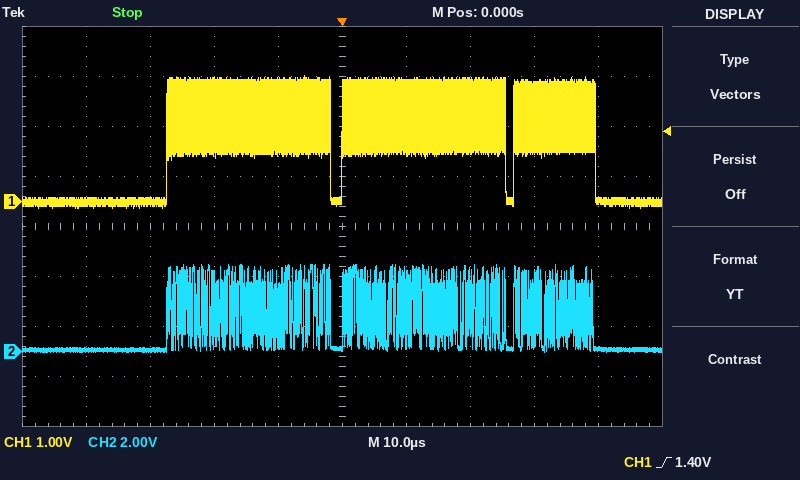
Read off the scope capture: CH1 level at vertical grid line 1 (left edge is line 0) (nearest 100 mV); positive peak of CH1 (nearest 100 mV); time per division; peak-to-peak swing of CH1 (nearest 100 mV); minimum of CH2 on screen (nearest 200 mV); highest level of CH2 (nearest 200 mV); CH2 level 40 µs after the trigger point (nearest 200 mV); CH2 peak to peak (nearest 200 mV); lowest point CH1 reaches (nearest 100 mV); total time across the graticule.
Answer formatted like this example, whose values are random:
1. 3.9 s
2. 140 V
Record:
1. 0.0 V
2. 2.5 V
3. 10 µs
4. 2.6 V
5. 0.0 V
6. 3.4 V
7. 200 mV
8. 3.4 V
9. -100 mV
10. 100 µs
